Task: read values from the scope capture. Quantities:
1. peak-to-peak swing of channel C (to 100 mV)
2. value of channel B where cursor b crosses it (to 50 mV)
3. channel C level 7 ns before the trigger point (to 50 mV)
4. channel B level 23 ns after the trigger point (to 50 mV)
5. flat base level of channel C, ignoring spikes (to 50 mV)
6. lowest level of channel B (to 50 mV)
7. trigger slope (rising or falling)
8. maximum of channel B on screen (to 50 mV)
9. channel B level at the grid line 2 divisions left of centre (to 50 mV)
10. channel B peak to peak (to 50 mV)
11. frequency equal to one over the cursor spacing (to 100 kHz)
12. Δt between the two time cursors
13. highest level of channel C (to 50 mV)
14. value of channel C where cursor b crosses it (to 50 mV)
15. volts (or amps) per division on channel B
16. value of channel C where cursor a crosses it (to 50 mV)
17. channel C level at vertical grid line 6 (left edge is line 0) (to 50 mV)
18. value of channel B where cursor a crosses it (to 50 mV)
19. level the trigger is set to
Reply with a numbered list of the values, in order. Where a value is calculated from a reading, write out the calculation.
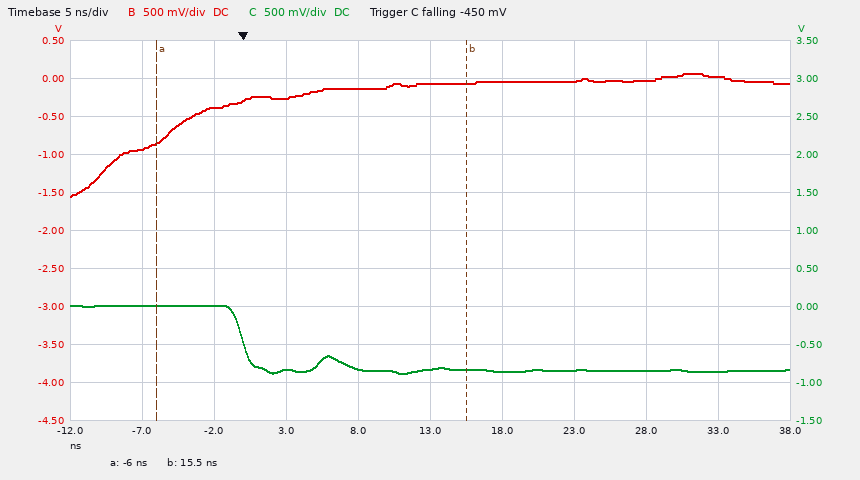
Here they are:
1. 900 mV
2. -50 mV
3. 0 mV
4. -50 mV
5. -850 mV
6. -1.55 V
7. falling
8. 50 mV
9. -250 mV
10. 50 mV − (-1.55 V) = 1.60 V
11. 1 / 21.5 ns ≈ 46.5 MHz
12. 15.5 ns − (-6 ns) = 21.5 ns
13. 0 mV
14. -850 mV
15. 500 mV
16. 0 mV
17. -850 mV
18. -850 mV
19. -450 mV
